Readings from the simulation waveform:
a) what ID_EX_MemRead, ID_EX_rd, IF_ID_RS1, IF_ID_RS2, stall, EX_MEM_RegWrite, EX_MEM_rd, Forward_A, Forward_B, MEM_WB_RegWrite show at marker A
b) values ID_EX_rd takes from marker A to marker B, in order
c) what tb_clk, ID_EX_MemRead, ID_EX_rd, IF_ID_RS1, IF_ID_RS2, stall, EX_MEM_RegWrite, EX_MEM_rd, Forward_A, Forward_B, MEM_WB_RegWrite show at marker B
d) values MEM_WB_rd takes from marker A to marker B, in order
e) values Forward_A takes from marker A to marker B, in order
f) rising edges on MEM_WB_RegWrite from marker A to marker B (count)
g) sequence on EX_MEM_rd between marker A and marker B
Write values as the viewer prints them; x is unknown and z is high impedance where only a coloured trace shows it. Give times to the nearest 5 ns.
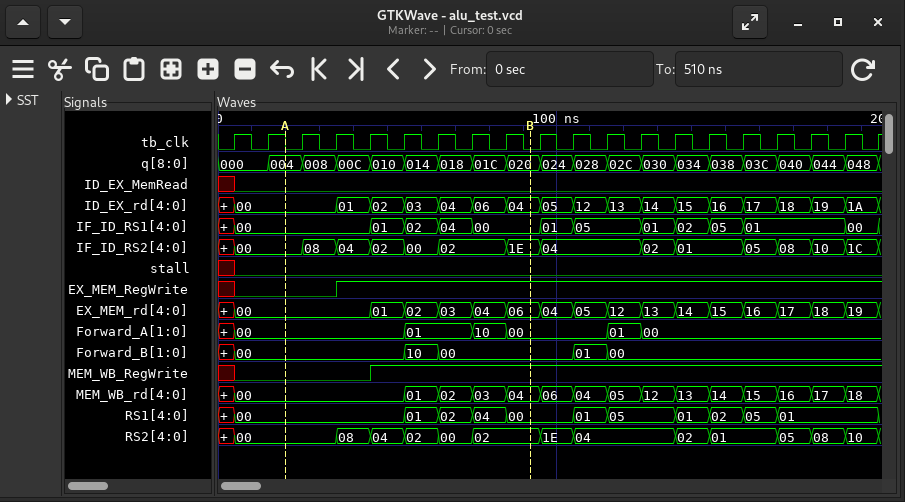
ID_EX_MemRead=0, ID_EX_rd=00, IF_ID_RS1=00, IF_ID_RS2=00, stall=0, EX_MEM_RegWrite=0, EX_MEM_rd=00, Forward_A=00, Forward_B=00, MEM_WB_RegWrite=0
00, 01, 02, 03, 04, 06, 04
tb_clk=0, ID_EX_MemRead=0, ID_EX_rd=04, IF_ID_RS1=00, IF_ID_RS2=1E, stall=0, EX_MEM_RegWrite=1, EX_MEM_rd=06, Forward_A=00, Forward_B=00, MEM_WB_RegWrite=1
00, 01, 02, 03, 04
00, 01, 10, 00
1
00, 01, 02, 03, 04, 06
